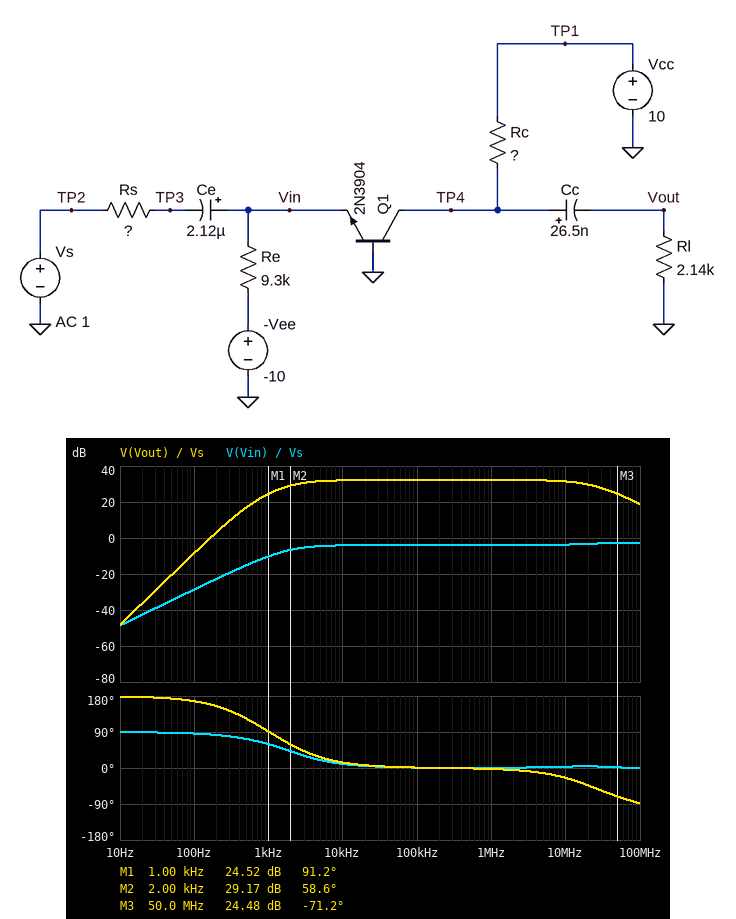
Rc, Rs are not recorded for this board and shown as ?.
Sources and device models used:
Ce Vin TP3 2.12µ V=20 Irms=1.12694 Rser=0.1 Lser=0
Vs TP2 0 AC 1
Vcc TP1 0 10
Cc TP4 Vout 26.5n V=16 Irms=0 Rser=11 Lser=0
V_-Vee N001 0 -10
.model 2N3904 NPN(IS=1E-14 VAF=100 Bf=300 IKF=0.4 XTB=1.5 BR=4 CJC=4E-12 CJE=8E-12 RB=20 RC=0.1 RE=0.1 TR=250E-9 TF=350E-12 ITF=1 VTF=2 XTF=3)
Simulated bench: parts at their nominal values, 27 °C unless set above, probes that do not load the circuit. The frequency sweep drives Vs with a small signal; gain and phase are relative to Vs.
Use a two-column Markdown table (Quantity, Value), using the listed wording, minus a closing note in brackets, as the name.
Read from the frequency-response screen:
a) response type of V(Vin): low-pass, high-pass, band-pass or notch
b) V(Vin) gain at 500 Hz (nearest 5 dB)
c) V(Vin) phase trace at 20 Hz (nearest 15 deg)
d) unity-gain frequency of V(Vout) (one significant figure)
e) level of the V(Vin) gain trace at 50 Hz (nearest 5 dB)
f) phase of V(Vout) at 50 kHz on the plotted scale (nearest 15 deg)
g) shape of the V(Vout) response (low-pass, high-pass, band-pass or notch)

| Quantity | Value |
|---|---|
| response type of V(Vin): low-pass, high-pass, band-pass or notch | high-pass |
| V(Vin) gain at 500 Hz | -15 dB |
| V(Vin) phase trace at 20 Hz | 90 deg |
| unity-gain frequency of V(Vout) | 200 Hz |
| level of the V(Vin) gain trace at 50 Hz | -35 dB |
| phase of V(Vout) at 50 kHz on the plotted scale | 0 deg |
| shape of the V(Vout) response | band-pass |
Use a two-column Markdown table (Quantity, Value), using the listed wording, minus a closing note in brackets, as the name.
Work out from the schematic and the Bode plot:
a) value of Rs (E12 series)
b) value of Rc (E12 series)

| Quantity | Value |
|---|---|
| value of Rs | 15 Ω |
| value of Rc | 8.2 kΩ |
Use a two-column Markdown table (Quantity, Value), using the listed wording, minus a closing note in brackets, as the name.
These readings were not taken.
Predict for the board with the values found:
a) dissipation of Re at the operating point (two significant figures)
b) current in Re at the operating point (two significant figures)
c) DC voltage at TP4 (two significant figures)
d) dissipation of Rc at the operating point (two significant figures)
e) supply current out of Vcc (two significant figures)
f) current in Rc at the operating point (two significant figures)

| Quantity | Value |
|---|---|
| dissipation of Re at the operating point | 9.4 mW |
| current in Re at the operating point | 1.0 mA |
| DC voltage at TP4 | 1.8 V |
| dissipation of Rc at the operating point | 8.2 mW |
| supply current out of Vcc | 1.0 mA |
| current in Rc at the operating point | 1.0 mA |
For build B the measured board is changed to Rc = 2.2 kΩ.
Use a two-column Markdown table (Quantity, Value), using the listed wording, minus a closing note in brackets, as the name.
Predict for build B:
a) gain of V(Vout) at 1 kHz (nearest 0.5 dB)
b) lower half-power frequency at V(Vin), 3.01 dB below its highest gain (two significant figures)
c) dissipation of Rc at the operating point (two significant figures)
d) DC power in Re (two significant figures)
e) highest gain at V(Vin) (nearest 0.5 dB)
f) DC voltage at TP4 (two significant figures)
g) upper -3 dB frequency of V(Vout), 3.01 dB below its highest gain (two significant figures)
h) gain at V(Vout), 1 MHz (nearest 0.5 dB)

| Quantity | Value |
|---|---|
| gain of V(Vout) at 1 kHz | 17.5 dB |
| lower half-power frequency at V(Vin), 3.01 dB below its highest gain | 2.5 kHz |
| dissipation of Rc at the operating point | 2.2 mW |
| DC power in Re | 9.4 mW |
| highest gain at V(Vin) | -3.0 dB |
| DC voltage at TP4 | 7.8 V |
| upper -3 dB frequency of V(Vout), 3.01 dB below its highest gain | 50 MHz |
| gain at V(Vout), 1 MHz | 28.5 dB |
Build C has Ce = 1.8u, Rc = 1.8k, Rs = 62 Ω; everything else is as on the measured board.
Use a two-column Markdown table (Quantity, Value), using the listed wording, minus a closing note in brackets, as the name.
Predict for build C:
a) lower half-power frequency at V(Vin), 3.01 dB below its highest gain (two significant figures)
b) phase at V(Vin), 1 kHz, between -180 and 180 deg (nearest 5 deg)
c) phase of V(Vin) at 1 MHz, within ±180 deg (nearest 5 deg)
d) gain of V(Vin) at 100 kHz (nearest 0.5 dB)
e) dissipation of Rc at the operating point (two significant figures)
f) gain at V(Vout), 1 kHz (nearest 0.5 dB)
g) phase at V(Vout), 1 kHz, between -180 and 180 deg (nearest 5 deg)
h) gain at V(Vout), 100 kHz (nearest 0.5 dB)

| Quantity | Value |
|---|---|
| lower half-power frequency at V(Vin), 3.01 dB below its highest gain | 2.2 kHz |
| phase at V(Vin), 1 kHz, between -180 and 180 deg | 45 deg |
| phase of V(Vin) at 1 MHz, within ±180 deg | 0 deg |
| gain of V(Vin) at 100 kHz | -10.5 dB |
| dissipation of Rc at the operating point | 1.8 mW |
| gain at V(Vout), 1 kHz | 12.5 dB |
| phase at V(Vout), 1 kHz, between -180 and 180 deg | 100 deg |
| gain at V(Vout), 100 kHz | 21.0 dB |
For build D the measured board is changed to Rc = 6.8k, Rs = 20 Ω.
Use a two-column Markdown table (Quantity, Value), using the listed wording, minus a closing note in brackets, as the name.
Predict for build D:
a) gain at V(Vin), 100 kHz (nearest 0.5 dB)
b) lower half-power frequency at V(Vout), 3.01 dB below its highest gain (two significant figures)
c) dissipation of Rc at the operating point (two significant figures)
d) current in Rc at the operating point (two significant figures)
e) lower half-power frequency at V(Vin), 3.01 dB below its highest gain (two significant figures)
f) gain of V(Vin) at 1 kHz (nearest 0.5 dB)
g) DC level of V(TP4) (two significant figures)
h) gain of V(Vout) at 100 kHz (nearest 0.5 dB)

| Quantity | Value |
|---|---|
| gain at V(Vin), 100 kHz | -5.0 dB |
| lower half-power frequency at V(Vout), 3.01 dB below its highest gain | 1.9 kHz |
| dissipation of Rc at the operating point | 6.8 mW |
| current in Rc at the operating point | 1.0 mA |
| lower half-power frequency at V(Vin), 3.01 dB below its highest gain | 2.5 kHz |
| gain of V(Vin) at 1 kHz | -10.5 dB |
| DC level of V(TP4) | 3.2 V |
| gain of V(Vout) at 100 kHz | 31.0 dB |
